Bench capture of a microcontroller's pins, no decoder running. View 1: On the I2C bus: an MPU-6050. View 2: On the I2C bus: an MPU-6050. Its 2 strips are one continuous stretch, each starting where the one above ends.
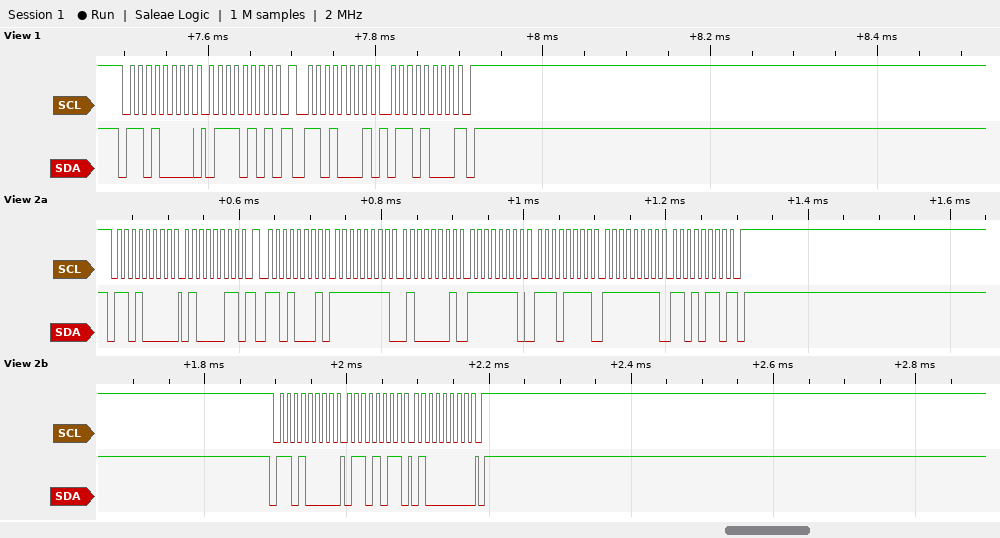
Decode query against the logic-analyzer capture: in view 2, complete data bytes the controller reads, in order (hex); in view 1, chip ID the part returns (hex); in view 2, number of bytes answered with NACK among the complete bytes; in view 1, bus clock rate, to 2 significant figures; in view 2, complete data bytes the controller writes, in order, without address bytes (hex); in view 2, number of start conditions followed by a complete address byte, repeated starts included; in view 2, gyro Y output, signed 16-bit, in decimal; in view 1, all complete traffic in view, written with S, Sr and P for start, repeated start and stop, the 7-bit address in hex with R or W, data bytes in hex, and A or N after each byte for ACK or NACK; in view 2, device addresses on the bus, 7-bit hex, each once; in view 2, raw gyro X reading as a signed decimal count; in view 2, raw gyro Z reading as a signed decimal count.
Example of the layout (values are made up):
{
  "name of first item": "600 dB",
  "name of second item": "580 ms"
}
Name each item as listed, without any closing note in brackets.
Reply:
{
  "in view 2, complete data bytes the controller reads, in order": "FF 41 FE EF FF D6",
  "in view 1, chip ID the part returns": "0x68",
  "in view 2, number of bytes answered with NACK among the complete bytes": "1",
  "in view 1, bus clock rate, to 2 significant figures": "100 kHz",
  "in view 2, complete data bytes the controller writes, in order, without address bytes": "43 6B 40",
  "in view 2, number of start conditions followed by a complete address byte, repeated starts included": "3",
  "in view 2, gyro Y output, signed 16-bit, in decimal": "-273",
  "in view 1, all complete traffic in view, written with S, Sr and P for start, repeated start and stop, the 7-bit address in hex with R or W, data bytes in hex, and A or N after each byte for ACK or NACK": "S 68W A 75 A Sr 68R A 68 N P",
  "in view 2, device addresses on the bus, 7-bit hex, each once": "0x68",
  "in view 2, raw gyro X reading as a signed decimal count": "-191",
  "in view 2, raw gyro Z reading as a signed decimal count": "-42"
}
